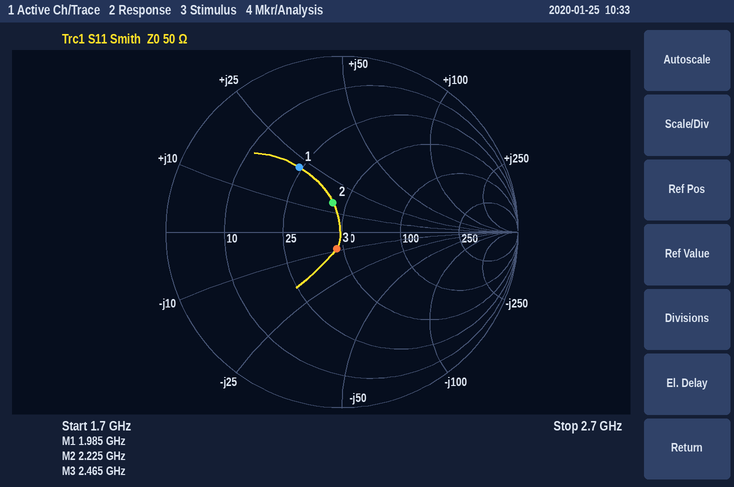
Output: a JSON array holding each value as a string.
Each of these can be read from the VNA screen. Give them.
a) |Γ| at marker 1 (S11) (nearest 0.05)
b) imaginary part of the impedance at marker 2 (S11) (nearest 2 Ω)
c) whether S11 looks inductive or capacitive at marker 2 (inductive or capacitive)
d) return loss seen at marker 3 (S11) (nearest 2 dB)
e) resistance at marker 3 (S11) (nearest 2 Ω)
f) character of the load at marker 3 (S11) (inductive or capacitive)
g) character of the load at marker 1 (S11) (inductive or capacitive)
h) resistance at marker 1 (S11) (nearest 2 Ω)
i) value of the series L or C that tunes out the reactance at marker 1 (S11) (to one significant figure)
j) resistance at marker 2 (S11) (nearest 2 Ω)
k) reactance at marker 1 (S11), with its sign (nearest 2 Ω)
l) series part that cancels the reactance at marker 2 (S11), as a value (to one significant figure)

["0.45", "+14 Ω", "inductive", "20 dB", "46 Ω", "capacitive", "inductive", "24 Ω", "4 pF", "42 Ω", "+22 Ω", "5 pF"]
